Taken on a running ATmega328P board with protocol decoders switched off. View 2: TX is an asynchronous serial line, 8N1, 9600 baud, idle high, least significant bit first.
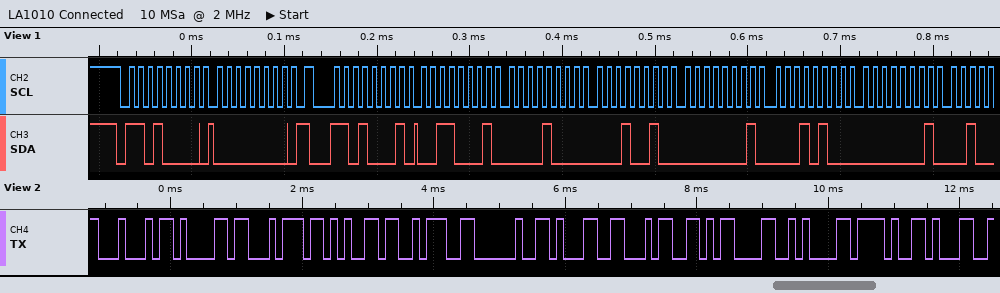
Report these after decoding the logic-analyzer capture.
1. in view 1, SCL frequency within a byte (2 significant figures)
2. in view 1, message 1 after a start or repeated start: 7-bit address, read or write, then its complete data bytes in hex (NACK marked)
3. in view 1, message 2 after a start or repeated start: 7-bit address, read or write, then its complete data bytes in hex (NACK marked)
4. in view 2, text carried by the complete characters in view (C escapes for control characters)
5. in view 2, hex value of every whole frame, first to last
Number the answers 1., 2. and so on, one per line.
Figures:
1. 100 kHz
2. 0x68 write: 00
3. 0x68 read: 31 08 12 01 14 01
4. "Date: 14\r\n/1"
5. 44 61 74 65 3A 20 31 34 0D 0A 2F 31
